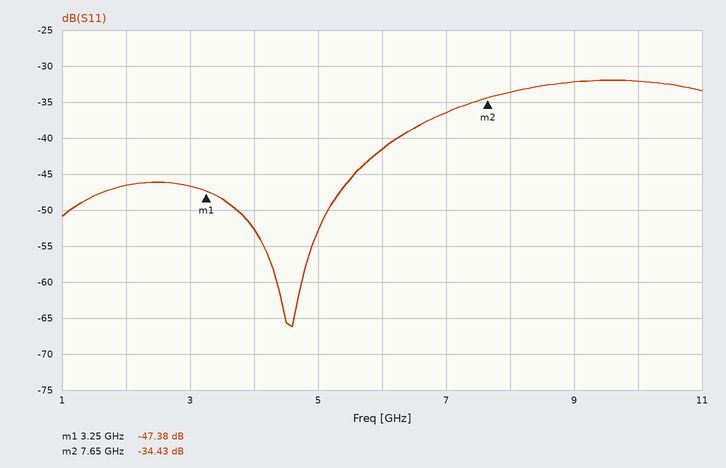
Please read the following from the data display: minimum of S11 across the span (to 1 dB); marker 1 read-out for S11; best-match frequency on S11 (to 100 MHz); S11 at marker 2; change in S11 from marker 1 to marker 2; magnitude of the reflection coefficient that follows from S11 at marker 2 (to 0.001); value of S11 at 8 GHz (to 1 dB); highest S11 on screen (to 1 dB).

-66 dB
-47.38 dB
4.6 GHz
-34.43 dB
12.95 dB
0.019
-34 dB
-32 dB
